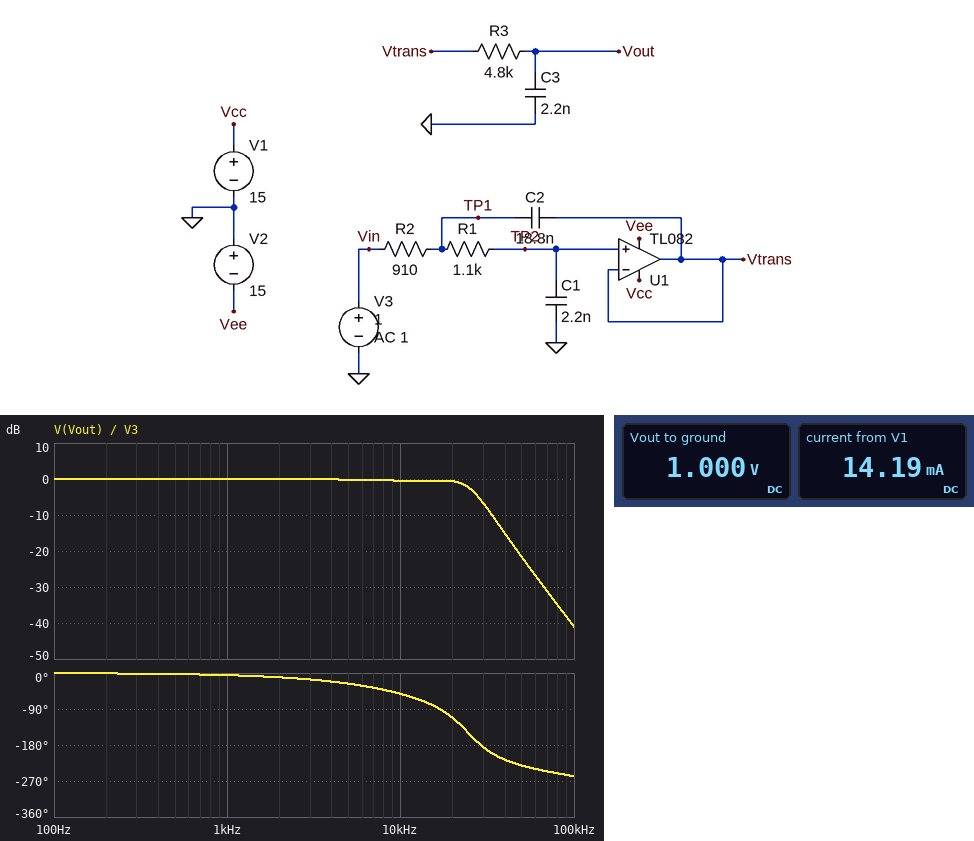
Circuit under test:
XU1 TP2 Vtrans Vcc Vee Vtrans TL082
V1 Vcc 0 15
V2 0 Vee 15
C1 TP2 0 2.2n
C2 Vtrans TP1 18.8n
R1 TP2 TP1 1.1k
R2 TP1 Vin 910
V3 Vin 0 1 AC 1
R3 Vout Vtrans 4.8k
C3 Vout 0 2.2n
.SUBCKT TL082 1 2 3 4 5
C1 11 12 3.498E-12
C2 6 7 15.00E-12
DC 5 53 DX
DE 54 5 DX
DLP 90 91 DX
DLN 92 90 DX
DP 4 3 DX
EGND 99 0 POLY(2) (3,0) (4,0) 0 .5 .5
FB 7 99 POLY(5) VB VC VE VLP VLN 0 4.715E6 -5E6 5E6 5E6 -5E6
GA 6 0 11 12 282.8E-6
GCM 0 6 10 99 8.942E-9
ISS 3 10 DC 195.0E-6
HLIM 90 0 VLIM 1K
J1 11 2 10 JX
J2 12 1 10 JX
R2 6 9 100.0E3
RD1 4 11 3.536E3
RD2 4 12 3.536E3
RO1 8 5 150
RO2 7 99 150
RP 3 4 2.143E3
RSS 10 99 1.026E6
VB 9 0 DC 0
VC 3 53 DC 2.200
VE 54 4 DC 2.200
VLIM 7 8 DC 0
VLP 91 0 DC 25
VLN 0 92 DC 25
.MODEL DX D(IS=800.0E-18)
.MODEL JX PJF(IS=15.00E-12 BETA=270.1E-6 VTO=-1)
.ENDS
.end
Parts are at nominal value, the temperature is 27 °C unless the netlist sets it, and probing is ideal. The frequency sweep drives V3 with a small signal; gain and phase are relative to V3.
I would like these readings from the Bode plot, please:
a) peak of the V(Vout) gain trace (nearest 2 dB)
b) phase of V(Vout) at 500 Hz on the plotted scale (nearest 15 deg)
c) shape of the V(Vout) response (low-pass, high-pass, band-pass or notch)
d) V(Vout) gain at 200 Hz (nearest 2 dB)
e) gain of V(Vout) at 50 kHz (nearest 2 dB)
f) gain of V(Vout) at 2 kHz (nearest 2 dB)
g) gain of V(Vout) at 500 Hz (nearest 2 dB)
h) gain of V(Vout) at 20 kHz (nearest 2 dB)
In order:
0 dB
0 deg
low-pass
0 dB
-22 dB
0 dB
0 dB
0 dB
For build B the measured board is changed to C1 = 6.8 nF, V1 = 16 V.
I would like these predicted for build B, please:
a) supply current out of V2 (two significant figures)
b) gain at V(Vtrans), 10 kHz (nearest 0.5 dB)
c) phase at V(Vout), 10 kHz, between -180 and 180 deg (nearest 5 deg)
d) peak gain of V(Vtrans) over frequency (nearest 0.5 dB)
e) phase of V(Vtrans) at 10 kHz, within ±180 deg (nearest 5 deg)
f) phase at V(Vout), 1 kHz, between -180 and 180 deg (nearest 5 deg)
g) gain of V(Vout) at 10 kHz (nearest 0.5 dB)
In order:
15 mA
0 dB
-95 deg
0.5 dB
-60 deg
-10 deg
-1.5 dB
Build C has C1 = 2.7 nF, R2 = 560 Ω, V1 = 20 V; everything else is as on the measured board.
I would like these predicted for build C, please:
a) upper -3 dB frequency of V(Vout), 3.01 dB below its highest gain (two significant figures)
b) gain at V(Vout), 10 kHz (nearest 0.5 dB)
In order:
25 kHz
-1.0 dB
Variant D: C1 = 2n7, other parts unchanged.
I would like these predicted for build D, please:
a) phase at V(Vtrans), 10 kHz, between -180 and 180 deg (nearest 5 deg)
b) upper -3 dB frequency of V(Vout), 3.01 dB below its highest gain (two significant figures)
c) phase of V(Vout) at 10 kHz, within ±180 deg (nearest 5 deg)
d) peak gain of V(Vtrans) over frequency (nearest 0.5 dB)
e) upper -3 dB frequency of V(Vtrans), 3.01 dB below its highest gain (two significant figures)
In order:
-25 deg
23 kHz
-55 deg
3.0 dB
26 kHz
